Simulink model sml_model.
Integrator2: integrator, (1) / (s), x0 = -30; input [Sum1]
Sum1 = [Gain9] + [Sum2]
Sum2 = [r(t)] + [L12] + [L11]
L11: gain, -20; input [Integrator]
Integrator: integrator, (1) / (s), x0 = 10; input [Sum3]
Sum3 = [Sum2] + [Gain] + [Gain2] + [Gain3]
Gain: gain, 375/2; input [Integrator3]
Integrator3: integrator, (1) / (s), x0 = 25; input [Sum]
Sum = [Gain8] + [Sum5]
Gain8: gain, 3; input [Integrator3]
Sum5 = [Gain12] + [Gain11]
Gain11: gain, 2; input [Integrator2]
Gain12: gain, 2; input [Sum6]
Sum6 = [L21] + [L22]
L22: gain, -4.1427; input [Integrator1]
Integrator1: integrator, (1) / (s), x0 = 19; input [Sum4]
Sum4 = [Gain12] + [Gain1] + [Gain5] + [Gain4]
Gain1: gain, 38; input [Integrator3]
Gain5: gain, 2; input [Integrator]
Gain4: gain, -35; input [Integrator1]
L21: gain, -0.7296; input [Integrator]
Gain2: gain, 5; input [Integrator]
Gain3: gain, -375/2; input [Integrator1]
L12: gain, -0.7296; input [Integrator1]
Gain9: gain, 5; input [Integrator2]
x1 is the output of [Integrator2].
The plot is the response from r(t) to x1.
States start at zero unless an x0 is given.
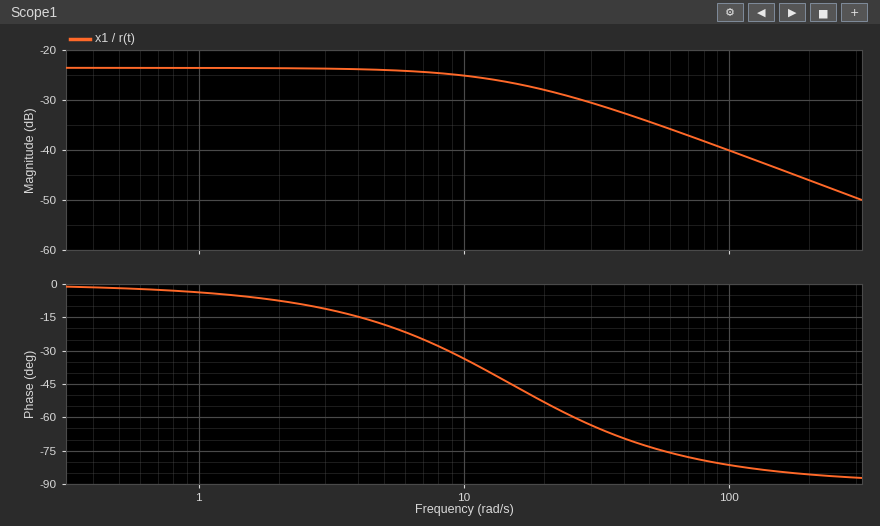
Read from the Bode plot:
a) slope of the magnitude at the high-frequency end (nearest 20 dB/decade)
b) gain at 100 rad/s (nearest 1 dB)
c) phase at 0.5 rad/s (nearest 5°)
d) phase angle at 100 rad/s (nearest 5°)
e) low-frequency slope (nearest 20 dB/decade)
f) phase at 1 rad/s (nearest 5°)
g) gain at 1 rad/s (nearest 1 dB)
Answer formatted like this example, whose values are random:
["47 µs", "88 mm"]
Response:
["-20 dB/decade", "-40 dB", "0°", "-80°", "0 dB/decade", "-5°", "-24 dB"]
